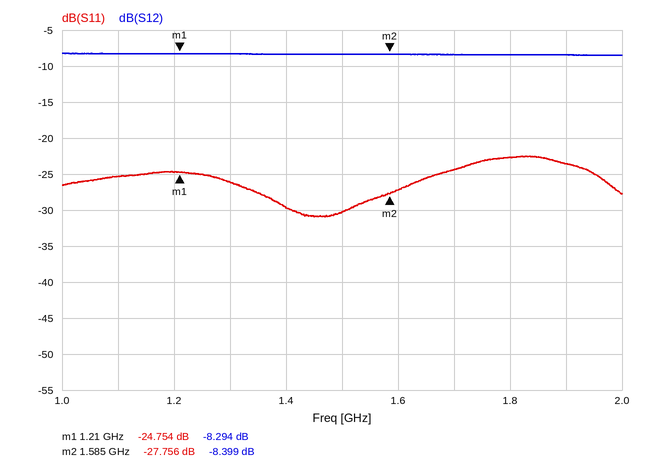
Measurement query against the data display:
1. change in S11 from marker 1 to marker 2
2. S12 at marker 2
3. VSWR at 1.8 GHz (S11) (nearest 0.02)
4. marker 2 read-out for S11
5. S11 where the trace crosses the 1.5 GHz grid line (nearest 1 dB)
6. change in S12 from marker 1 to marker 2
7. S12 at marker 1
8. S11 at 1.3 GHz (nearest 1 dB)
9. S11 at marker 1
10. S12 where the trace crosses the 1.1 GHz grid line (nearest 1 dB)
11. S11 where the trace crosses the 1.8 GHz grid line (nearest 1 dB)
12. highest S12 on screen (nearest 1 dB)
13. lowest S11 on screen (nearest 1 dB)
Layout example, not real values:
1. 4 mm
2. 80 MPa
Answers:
1. -3.002 dB
2. -8.399 dB
3. 1.16
4. -27.756 dB
5. -30 dB
6. -0.105 dB
7. -8.294 dB
8. -26 dB
9. -24.754 dB
10. -8 dB
11. -23 dB
12. -8 dB
13. -31 dB
